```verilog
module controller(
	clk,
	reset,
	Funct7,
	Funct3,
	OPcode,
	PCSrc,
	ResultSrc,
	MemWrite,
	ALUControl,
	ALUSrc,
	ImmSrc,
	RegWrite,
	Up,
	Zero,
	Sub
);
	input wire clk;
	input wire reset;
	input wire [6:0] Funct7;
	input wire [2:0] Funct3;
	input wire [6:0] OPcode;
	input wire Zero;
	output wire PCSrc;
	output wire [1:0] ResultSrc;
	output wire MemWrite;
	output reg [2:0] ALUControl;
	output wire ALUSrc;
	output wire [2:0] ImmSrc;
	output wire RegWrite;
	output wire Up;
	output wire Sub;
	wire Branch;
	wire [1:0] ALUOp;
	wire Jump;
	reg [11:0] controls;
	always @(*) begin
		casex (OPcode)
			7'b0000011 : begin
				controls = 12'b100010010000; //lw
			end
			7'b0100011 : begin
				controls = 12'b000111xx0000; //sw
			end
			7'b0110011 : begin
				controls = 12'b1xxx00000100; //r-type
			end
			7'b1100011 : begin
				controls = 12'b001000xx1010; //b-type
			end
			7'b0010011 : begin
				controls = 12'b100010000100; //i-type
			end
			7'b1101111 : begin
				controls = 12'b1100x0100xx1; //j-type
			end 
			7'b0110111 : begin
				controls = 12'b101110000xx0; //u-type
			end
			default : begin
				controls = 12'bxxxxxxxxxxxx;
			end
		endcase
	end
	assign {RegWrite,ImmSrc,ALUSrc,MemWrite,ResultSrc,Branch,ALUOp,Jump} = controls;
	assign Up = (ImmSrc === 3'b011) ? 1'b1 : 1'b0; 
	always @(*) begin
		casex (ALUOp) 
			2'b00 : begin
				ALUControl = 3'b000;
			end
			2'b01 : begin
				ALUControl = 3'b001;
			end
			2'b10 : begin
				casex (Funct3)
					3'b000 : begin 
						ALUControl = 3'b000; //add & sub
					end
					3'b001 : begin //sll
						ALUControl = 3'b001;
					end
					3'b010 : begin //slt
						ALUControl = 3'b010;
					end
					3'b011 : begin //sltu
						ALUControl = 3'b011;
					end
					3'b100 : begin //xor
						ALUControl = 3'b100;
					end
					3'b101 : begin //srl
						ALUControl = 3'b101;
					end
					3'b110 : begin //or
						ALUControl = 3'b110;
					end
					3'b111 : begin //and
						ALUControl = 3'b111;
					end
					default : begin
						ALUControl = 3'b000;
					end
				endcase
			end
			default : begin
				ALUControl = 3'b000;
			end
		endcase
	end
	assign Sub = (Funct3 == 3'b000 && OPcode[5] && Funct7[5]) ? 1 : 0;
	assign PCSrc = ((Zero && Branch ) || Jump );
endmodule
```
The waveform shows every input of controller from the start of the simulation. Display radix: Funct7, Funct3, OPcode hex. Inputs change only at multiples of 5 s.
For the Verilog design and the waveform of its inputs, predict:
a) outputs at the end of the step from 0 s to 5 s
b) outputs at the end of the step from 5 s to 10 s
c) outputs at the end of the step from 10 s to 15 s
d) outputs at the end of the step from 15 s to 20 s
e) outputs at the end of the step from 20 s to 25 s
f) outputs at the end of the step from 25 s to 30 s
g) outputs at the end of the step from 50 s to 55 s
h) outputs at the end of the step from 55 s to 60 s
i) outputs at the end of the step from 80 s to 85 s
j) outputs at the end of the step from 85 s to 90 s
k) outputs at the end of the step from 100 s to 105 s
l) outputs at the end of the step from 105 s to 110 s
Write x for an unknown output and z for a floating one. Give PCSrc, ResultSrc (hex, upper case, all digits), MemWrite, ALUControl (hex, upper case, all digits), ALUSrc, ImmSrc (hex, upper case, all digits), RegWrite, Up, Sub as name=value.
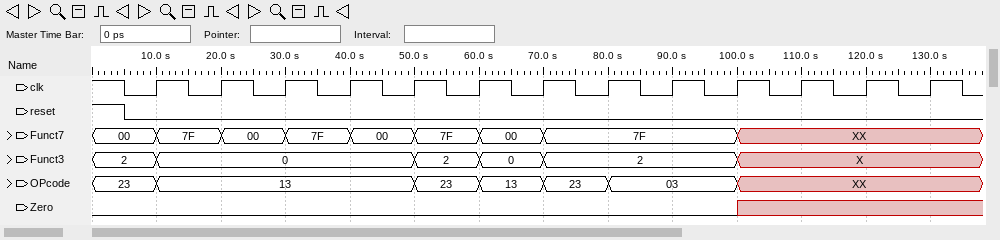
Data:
PCSrc=0, ResultSrc=x, MemWrite=1, ALUControl=0, ALUSrc=1, ImmSrc=1, RegWrite=0, Up=0, Sub=0
PCSrc=0, ResultSrc=x, MemWrite=1, ALUControl=0, ALUSrc=1, ImmSrc=1, RegWrite=0, Up=0, Sub=0
PCSrc=0, ResultSrc=0, MemWrite=0, ALUControl=0, ALUSrc=1, ImmSrc=0, RegWrite=1, Up=0, Sub=0
PCSrc=0, ResultSrc=0, MemWrite=0, ALUControl=0, ALUSrc=1, ImmSrc=0, RegWrite=1, Up=0, Sub=0
PCSrc=0, ResultSrc=0, MemWrite=0, ALUControl=0, ALUSrc=1, ImmSrc=0, RegWrite=1, Up=0, Sub=0
PCSrc=0, ResultSrc=0, MemWrite=0, ALUControl=0, ALUSrc=1, ImmSrc=0, RegWrite=1, Up=0, Sub=0
PCSrc=0, ResultSrc=x, MemWrite=1, ALUControl=0, ALUSrc=1, ImmSrc=1, RegWrite=0, Up=0, Sub=0
PCSrc=0, ResultSrc=x, MemWrite=1, ALUControl=0, ALUSrc=1, ImmSrc=1, RegWrite=0, Up=0, Sub=0
PCSrc=0, ResultSrc=1, MemWrite=0, ALUControl=0, ALUSrc=1, ImmSrc=0, RegWrite=1, Up=0, Sub=0
PCSrc=0, ResultSrc=1, MemWrite=0, ALUControl=0, ALUSrc=1, ImmSrc=0, RegWrite=1, Up=0, Sub=0
PCSrc=0, ResultSrc=1, MemWrite=0, ALUControl=0, ALUSrc=1, ImmSrc=0, RegWrite=1, Up=0, Sub=x
PCSrc=0, ResultSrc=1, MemWrite=0, ALUControl=0, ALUSrc=1, ImmSrc=0, RegWrite=1, Up=0, Sub=x
